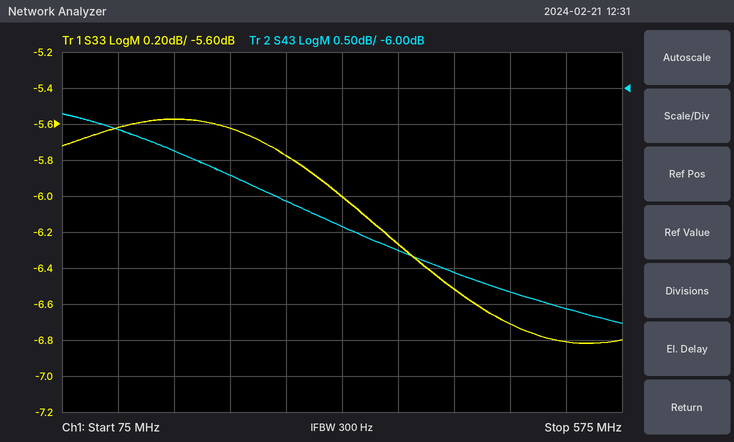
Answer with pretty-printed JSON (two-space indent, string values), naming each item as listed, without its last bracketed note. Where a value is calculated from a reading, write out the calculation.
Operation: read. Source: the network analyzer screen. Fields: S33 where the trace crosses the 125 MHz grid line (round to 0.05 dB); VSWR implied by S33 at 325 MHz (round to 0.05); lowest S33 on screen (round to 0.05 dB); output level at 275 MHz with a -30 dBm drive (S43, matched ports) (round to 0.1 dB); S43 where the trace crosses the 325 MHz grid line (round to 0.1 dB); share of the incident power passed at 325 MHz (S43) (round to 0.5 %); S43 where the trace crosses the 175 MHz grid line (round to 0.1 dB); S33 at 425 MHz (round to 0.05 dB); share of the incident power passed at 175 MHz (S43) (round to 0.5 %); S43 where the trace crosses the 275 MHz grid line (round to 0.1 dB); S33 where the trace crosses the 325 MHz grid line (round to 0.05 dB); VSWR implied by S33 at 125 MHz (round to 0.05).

{
  "S33 where the trace crosses the 125 MHz grid line": "-5.60 dB",
  "VSWR implied by S33 at 325 MHz": "|Γ| = 10^(-6/20) = 0.5012; VSWR = (1 + 0.5012)/(1 − 0.5012) ≈ 3.01, so 3.00 to the nearest 0.05",
  "lowest S33 on screen": "-6.80 dB",
  "output level at 275 MHz with a -30 dBm drive (S43, matched ports)": "-30 dBm + (-7.6 dB) = -37.6 dBm",
  "S43 where the trace crosses the 325 MHz grid line": "-7.9 dB",
  "share of the incident power passed at 325 MHz (S43)": "10^(-7.9/10) ≈ 16.2 %, so 16.0 % to the nearest 0.5 %",
  "S43 where the trace crosses the 175 MHz grid line": "-6.9 dB",
  "S33 at 425 MHz": "-6.50 dB",
  "share of the incident power passed at 175 MHz (S43)": "10^(-6.9/10) ≈ 20.4 %, so 20.5 % to the nearest 0.5 %",
  "S43 where the trace crosses the 275 MHz grid line": "-7.6 dB",
  "S33 where the trace crosses the 325 MHz grid line": "-6.00 dB",
  "VSWR implied by S33 at 125 MHz": "|Γ| = 10^(-5.6/20) = 0.5248; VSWR = (1 + 0.5248)/(1 − 0.5248) ≈ 3.21, so 3.20 to the nearest 0.05"
}
